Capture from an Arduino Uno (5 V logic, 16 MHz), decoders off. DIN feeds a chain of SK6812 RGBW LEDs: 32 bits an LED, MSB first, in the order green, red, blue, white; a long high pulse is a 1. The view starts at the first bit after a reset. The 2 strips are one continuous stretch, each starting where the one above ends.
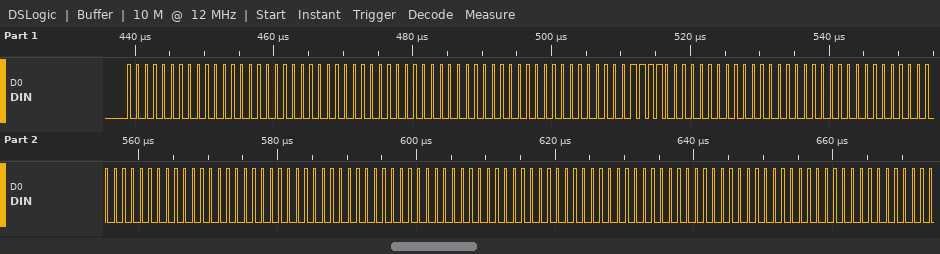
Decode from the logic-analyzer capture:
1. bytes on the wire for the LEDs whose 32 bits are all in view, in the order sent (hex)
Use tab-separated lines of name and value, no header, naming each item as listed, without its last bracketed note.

bytes on the wire for the LEDs whose 32 bits are all in view, in the order sent	00 00 00 00 00 00 00 3C 00 00 00 00 00 00 00 00 00 00 00 00
